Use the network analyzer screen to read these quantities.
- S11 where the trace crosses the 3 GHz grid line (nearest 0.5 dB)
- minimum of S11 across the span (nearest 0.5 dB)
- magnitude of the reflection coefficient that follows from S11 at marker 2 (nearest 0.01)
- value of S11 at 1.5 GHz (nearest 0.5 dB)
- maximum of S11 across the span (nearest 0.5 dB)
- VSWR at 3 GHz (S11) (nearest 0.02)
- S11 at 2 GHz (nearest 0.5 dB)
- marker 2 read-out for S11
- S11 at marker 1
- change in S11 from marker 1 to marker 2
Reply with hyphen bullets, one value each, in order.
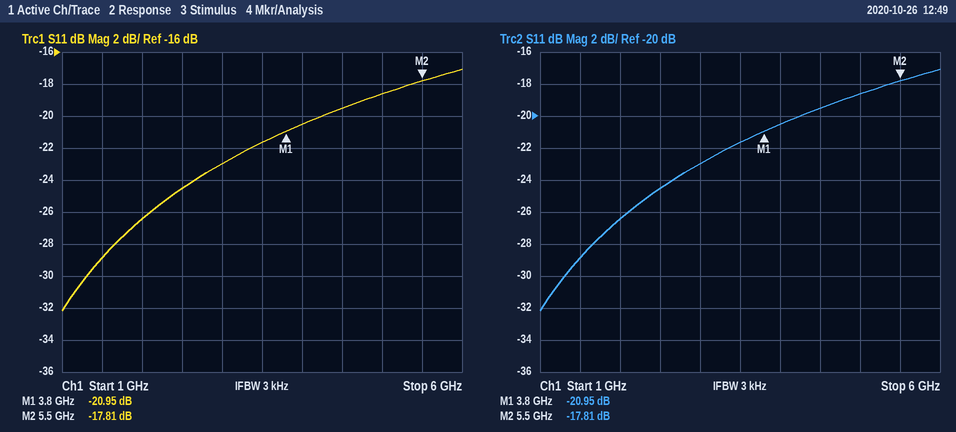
- -23.0 dB
- -32.0 dB
- 0.13
- -29.0 dB
- -17.0 dB
- 1.16
- -26.5 dB
- -17.81 dB
- -20.95 dB
- 3.14 dB
